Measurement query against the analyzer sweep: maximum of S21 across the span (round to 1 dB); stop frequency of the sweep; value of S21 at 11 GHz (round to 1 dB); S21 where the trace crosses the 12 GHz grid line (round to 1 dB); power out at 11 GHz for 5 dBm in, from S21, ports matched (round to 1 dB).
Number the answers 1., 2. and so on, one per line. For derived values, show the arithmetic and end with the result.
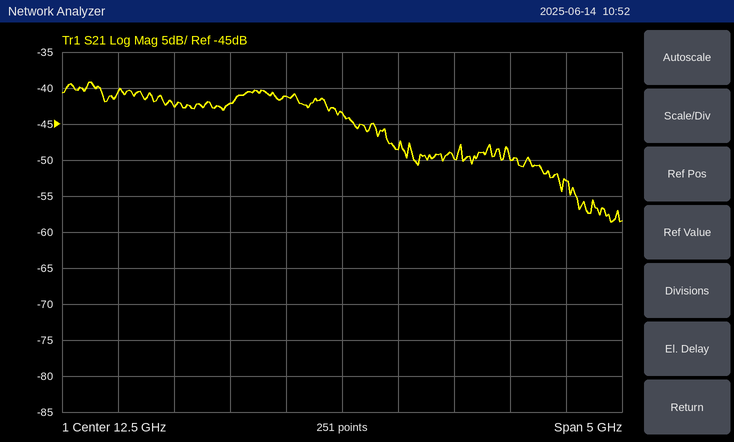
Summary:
1. -39 dB
2. 15 GHz
3. -43 dB
4. -41 dB
5. 5 dBm + (-43 dB) = -38 dBm
